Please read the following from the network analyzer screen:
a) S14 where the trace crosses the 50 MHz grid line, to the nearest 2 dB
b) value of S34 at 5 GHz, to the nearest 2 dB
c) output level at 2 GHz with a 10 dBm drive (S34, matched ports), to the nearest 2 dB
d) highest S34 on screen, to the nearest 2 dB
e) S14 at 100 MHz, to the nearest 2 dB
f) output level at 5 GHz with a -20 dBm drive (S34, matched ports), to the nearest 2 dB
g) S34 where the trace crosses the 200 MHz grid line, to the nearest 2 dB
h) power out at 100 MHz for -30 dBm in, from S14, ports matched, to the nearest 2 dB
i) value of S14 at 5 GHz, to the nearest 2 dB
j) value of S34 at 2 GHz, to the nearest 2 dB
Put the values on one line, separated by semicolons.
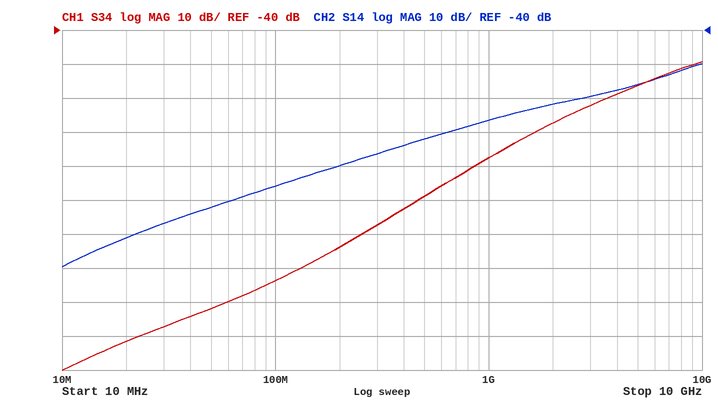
-92 dB; -56 dB; -58 dBm; -50 dB; -86 dB; -76 dBm; -104 dB; -116 dBm; -56 dB; -68 dB
